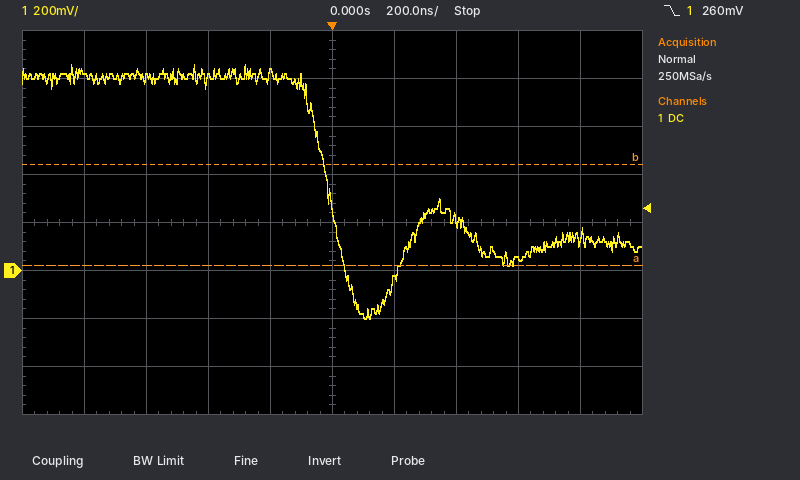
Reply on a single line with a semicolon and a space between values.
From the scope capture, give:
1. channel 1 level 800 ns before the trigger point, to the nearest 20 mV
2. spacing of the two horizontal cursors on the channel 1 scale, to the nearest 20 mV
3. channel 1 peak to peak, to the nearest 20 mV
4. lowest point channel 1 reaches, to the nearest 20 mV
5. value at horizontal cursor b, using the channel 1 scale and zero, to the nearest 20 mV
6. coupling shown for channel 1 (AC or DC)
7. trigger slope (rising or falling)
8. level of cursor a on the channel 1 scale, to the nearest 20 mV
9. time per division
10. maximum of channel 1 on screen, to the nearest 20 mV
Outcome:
820 mV; 420 mV; 1.06 V; -200 mV; 440 mV; DC; falling; 20 mV; 200 ns; 860 mV
